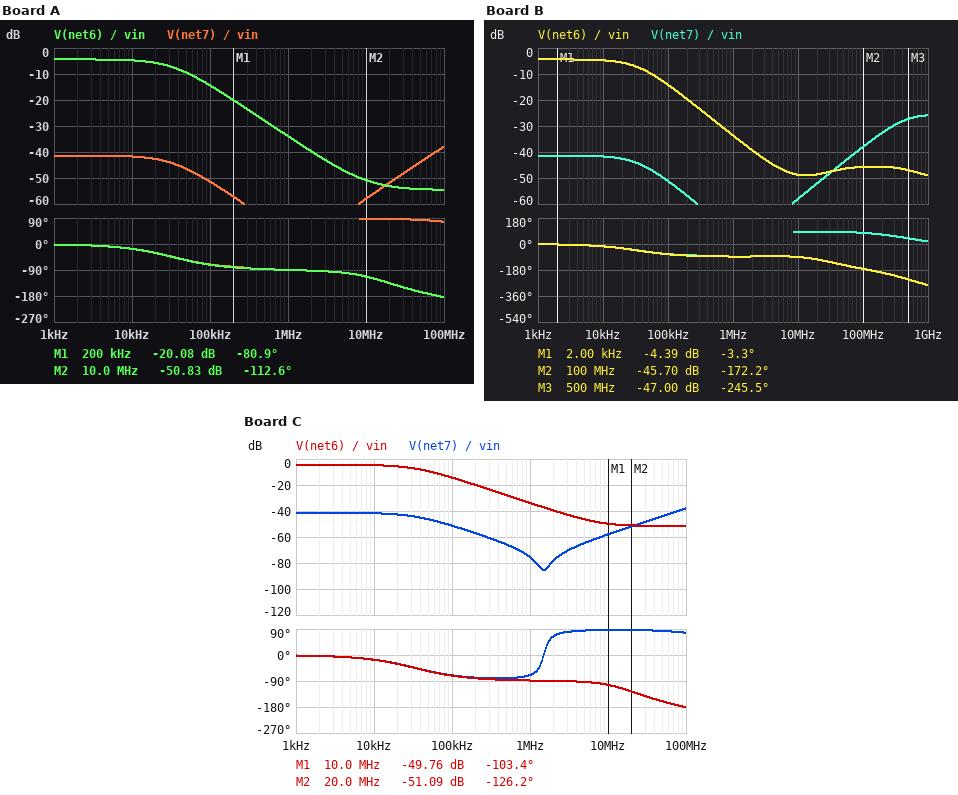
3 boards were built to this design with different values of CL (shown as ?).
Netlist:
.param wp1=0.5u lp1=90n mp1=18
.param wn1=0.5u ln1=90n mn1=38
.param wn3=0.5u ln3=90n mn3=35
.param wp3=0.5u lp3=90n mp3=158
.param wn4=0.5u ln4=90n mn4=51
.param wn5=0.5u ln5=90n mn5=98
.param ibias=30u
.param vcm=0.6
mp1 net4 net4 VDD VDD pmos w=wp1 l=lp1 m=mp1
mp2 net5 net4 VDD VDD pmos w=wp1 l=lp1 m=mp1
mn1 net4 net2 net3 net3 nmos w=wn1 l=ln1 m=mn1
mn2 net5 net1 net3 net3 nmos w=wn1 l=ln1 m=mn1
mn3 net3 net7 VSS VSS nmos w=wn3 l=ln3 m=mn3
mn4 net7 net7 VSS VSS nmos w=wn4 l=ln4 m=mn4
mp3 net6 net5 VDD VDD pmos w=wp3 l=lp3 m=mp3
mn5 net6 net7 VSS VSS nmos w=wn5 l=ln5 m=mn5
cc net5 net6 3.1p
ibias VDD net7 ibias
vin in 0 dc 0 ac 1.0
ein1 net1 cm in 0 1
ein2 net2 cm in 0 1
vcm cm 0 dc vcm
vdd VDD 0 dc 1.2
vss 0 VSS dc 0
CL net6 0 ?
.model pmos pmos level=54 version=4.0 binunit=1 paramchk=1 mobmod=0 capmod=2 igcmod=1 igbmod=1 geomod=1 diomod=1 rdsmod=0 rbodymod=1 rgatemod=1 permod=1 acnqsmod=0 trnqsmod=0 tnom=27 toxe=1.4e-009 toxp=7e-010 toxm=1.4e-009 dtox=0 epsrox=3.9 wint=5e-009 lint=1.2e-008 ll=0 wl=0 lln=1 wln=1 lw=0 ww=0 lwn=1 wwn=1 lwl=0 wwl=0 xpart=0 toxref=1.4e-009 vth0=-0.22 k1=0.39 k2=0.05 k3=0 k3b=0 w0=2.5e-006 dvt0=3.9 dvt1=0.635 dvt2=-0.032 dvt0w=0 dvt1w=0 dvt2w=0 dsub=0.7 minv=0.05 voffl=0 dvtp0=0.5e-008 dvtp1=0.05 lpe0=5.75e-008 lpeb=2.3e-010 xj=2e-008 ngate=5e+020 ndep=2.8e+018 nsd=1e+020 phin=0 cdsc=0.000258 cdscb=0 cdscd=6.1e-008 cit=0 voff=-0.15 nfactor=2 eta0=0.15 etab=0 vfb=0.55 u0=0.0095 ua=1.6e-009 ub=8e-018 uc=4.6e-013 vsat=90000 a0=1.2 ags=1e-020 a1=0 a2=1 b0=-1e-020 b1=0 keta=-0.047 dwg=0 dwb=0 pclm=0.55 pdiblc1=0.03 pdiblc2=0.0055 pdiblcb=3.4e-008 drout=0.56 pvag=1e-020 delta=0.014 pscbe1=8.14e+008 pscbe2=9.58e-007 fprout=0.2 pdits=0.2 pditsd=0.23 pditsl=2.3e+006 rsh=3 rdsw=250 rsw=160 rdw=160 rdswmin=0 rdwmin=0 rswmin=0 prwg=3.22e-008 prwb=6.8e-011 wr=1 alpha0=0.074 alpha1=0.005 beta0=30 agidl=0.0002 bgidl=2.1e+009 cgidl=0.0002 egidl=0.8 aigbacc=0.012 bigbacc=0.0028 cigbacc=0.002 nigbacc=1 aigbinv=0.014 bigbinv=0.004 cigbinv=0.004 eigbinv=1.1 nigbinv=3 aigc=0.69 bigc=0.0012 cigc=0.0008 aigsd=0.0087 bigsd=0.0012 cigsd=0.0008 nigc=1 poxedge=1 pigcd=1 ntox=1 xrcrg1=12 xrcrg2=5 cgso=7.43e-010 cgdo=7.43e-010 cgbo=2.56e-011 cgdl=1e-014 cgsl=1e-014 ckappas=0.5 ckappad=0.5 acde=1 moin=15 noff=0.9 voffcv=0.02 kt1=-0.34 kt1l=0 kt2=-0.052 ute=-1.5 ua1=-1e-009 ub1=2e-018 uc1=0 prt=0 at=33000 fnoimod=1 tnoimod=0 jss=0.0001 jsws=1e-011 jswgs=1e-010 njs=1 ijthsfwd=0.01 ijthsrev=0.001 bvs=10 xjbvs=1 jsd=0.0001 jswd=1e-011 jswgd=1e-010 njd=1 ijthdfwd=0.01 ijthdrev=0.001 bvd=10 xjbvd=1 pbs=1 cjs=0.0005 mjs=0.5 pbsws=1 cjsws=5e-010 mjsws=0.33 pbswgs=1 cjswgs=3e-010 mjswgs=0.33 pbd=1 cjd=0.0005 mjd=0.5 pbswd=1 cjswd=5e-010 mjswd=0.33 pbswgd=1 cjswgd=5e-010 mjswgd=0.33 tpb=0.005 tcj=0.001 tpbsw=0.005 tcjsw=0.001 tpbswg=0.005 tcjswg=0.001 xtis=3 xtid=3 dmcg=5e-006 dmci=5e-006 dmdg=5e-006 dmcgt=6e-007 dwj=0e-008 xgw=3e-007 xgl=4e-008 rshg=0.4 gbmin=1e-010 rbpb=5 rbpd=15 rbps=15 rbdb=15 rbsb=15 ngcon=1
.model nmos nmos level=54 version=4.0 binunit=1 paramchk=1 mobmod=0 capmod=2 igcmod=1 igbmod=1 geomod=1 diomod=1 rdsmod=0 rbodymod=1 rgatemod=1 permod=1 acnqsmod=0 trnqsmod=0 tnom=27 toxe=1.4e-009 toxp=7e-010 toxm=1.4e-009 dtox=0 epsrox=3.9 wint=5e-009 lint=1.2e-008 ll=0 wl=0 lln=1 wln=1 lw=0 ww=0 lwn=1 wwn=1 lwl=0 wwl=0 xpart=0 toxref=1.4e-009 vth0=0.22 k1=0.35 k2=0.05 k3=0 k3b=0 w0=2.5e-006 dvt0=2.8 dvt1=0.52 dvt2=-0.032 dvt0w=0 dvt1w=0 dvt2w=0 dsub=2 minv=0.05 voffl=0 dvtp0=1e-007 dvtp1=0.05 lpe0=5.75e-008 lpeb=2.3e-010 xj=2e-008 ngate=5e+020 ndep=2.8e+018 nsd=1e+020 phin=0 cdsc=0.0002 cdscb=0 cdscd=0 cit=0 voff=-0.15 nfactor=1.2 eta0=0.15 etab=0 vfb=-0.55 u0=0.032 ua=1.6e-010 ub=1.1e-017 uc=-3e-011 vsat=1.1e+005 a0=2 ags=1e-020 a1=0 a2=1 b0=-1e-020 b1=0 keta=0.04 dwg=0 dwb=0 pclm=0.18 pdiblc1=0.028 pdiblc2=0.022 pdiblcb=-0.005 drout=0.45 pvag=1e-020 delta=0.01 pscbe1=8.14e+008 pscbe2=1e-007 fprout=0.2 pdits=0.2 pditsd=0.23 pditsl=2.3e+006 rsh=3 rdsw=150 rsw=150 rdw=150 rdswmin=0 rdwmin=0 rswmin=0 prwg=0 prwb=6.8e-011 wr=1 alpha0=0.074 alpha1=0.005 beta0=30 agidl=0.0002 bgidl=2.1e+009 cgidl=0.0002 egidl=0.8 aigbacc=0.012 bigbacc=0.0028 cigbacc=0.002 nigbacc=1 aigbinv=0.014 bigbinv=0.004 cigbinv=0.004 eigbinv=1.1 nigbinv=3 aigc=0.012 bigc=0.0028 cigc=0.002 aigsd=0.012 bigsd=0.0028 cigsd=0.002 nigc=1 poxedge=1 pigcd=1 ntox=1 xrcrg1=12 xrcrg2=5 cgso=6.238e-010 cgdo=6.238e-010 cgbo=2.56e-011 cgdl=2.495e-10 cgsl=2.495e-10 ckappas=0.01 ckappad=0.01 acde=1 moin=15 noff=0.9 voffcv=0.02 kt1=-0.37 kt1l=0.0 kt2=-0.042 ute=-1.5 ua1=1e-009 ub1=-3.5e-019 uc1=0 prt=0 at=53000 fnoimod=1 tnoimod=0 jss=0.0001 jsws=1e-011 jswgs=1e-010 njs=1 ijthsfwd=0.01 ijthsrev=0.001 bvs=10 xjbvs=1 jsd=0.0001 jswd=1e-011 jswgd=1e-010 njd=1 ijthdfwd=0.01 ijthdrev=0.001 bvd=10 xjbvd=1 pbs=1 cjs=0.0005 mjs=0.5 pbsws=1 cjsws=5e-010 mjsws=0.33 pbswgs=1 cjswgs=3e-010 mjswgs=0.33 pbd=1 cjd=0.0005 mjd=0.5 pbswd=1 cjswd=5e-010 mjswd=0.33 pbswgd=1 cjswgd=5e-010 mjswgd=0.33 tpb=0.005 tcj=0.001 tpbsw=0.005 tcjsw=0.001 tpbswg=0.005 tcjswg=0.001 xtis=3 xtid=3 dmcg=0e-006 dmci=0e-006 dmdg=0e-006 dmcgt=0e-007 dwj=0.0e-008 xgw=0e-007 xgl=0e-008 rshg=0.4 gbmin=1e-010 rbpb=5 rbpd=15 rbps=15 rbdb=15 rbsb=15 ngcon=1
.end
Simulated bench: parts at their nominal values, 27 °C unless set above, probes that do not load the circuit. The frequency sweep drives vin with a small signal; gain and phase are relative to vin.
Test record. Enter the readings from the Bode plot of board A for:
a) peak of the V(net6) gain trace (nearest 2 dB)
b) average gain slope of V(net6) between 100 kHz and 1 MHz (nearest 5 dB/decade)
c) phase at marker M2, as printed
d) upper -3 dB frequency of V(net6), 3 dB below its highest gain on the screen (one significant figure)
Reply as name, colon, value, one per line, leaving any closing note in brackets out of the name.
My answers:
peak of the V(net6) gain trace: -4 dB
average gain slope of V(net6) between 100 kHz and 1 MHz: -20 dB/decade
phase at marker M2, as printed: -112.6 deg
upper -3 dB frequency of V(net6), 3 dB below its highest gain on the screen: 30 kHz
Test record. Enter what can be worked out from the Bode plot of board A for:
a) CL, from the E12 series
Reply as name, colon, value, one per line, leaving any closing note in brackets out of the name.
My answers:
CL, from the E12 series: 22 pF
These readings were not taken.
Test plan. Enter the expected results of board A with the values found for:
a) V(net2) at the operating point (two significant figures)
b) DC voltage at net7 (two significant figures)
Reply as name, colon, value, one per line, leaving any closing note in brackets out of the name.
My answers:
V(net2) at the operating point: 600 mV
DC voltage at net7: 300 mV
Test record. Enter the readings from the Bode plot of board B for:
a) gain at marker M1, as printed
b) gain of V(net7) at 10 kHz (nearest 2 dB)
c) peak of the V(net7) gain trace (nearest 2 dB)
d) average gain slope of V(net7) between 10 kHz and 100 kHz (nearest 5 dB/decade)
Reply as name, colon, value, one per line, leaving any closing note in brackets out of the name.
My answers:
gain at marker M1, as printed: -4.39 dB
gain of V(net7) at 10 kHz: -42 dB
peak of the V(net7) gain trace: -26 dB
average gain slope of V(net7) between 10 kHz and 100 kHz: -10 dB/decade
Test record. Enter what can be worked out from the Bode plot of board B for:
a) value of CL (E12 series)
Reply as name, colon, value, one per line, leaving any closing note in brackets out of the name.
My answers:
value of CL: 6.8 pF
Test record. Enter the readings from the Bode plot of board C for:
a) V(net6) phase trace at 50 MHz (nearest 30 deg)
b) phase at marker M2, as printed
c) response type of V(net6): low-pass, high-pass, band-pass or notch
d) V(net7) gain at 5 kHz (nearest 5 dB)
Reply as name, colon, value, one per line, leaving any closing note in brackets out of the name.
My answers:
V(net6) phase trace at 50 MHz: -150 deg
phase at marker M2, as printed: -126.2 deg
response type of V(net6): low-pass, high-pass, band-pass or notch: low-pass
V(net7) gain at 5 kHz: -40 dB
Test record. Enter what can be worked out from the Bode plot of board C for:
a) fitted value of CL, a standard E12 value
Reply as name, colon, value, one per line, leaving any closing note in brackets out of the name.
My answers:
fitted value of CL, a standard E12 value: 15 pF
